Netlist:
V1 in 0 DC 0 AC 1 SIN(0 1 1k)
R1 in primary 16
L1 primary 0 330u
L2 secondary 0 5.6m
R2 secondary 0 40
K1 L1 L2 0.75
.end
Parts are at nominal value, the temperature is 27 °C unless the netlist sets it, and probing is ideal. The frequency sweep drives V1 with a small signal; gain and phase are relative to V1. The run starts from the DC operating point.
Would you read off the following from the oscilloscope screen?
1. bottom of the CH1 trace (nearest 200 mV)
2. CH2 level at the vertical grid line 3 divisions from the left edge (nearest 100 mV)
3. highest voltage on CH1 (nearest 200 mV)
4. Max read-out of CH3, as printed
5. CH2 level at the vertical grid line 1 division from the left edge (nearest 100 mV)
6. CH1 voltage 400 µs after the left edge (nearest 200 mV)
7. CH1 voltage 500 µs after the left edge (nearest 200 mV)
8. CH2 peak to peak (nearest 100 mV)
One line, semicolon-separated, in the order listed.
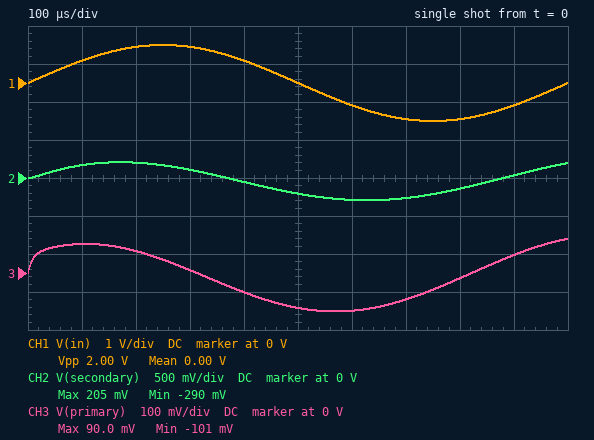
-1.0 V; 100 mV; 1.0 V; 90.0 mV; 200 mV; 600 mV; 0 V; 500 mV
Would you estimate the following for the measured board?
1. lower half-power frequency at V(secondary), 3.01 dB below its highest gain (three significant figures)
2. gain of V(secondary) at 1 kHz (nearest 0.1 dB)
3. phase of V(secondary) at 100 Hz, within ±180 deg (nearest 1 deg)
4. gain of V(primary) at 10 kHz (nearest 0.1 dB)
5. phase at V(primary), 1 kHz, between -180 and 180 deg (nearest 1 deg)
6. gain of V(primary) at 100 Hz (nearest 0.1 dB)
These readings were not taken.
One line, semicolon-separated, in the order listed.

947 Hz; -10.8 dB; 84 deg; -6.5 dB; 64 deg; -37.8 dB
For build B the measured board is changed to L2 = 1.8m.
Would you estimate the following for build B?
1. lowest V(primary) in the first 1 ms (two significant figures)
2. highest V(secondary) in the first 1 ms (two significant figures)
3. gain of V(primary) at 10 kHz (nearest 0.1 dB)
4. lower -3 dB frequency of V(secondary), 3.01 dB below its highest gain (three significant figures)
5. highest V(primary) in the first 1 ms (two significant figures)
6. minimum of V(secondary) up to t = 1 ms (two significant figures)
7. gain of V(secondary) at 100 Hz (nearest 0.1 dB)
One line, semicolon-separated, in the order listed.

-120 mV; 200 mV; -6.1 dB; 2.23 kHz; 120 mV; -210 mV; -32.9 dB
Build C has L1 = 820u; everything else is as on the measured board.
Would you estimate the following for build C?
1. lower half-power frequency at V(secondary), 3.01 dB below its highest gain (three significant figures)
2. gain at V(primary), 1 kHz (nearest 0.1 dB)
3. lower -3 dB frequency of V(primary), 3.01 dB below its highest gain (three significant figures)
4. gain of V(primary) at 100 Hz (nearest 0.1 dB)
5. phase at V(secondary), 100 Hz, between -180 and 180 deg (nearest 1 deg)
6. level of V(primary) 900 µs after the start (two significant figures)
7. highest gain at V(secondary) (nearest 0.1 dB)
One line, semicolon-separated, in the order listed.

771 Hz; -12.7 dB; 8.09 kHz; -29.9 dB; 83 deg; 83 mV; -5.6 dB
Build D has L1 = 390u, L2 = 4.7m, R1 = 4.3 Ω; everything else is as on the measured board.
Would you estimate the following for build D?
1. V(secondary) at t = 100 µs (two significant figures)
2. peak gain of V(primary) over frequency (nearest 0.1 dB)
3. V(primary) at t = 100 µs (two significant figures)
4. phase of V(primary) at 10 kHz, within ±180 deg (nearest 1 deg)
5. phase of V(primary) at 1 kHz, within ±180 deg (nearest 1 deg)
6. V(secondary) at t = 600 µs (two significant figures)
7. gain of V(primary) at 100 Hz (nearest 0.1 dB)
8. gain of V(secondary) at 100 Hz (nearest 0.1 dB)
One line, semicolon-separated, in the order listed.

470 mV; 0 dB; 270 mV; 20 deg; 50 deg; -920 mV; -24.9 dB; -16.6 dB
